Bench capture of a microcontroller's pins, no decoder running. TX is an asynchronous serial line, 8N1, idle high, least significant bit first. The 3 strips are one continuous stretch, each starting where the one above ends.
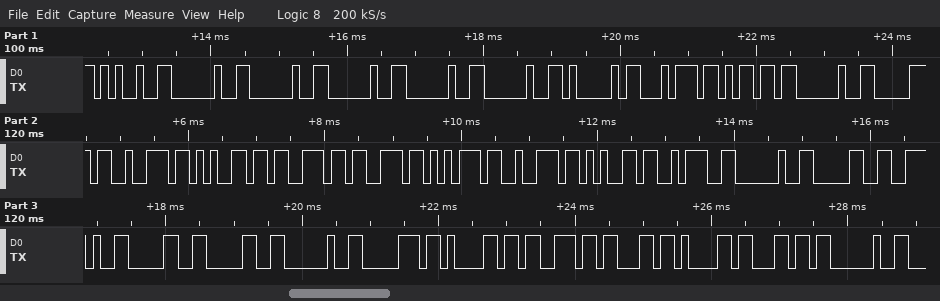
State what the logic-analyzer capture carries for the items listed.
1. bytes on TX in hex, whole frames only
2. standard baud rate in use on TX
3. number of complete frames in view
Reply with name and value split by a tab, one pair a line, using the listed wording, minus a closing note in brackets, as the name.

bytes on TX in hex, whole frames only	25 20 20 20 20 20 41 74 6D 20 70 72 65 73 73 75 72 65 3A 20 30 2E 30 30 20 70 61 73 63 61 6C 20
standard baud rate in use on TX	9600 baud
number of complete frames in view	32
